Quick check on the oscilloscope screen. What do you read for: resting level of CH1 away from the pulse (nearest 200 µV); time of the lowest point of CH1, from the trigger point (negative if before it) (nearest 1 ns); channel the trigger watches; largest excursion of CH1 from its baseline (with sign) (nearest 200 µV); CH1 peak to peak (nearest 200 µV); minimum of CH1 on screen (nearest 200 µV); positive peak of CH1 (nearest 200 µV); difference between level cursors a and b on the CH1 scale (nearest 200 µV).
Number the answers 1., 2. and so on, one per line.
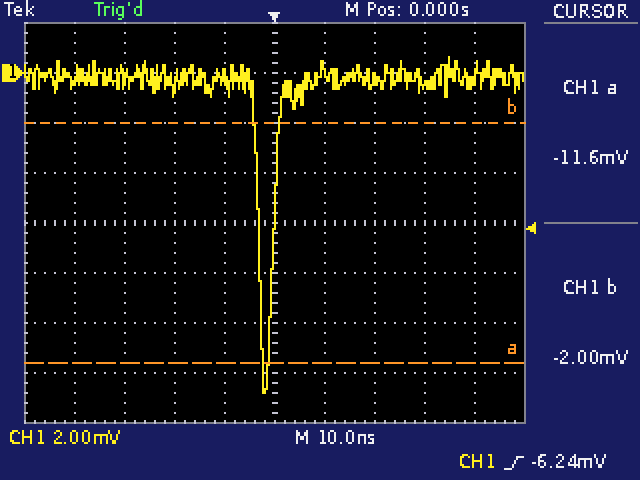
1. -200 µV
2. -2 ns
3. CH1
4. -12.6 mV
5. 13.4 mV
6. -12.8 mV
7. 600 µV
8. 9.6 mV
